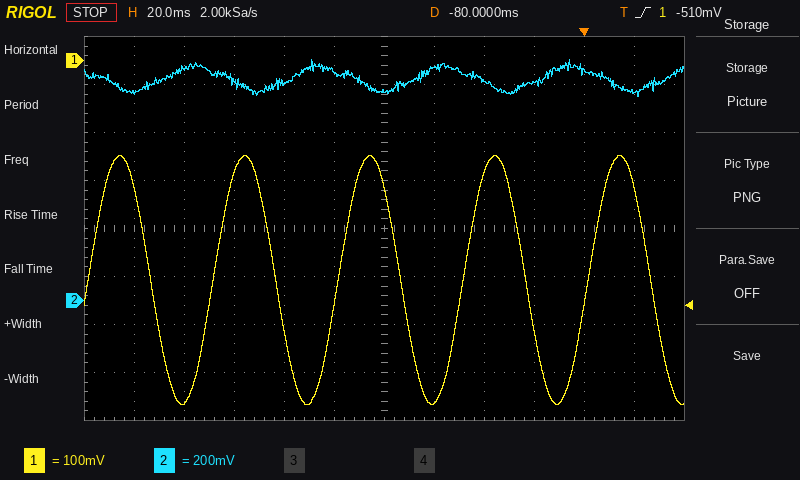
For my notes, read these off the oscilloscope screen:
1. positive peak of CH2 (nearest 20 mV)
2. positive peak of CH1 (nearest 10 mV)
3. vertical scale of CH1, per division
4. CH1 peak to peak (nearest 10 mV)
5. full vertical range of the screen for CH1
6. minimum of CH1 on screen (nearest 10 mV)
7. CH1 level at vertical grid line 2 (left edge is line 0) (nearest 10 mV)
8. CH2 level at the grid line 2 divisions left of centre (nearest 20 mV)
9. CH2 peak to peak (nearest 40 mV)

1.00 V
-200 mV
100 mV
520 mV
800 mV
-720 mV
-710 mV
900 mV
160 mV
